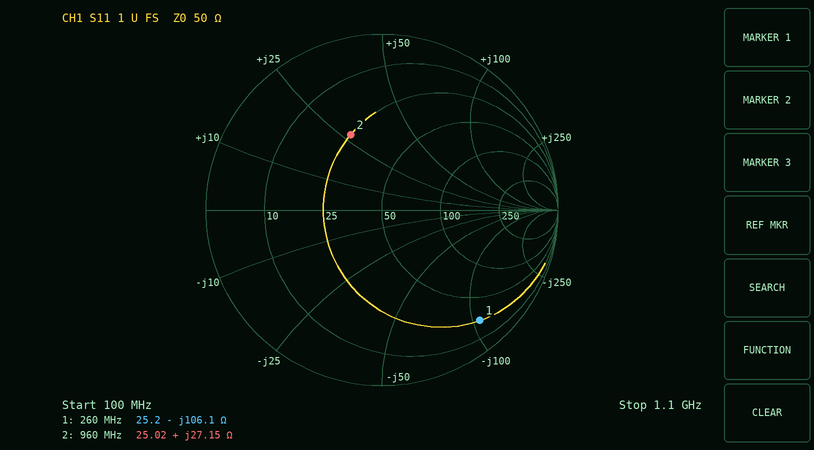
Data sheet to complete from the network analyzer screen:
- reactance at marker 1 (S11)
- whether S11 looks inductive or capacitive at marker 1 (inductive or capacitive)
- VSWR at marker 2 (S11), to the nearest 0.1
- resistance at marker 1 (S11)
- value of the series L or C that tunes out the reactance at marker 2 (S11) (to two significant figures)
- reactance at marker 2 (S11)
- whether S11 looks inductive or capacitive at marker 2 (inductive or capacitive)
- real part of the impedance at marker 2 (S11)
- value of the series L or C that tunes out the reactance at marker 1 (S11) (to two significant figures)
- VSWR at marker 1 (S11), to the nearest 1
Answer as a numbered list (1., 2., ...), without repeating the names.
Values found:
1. -106.1 Ω
2. capacitive
3. 2.7
4. 25.2 Ω
5. 6.1 pF
6. +27.15 Ω
7. inductive
8. 25.02 Ω
9. 65 nH
10. 11
